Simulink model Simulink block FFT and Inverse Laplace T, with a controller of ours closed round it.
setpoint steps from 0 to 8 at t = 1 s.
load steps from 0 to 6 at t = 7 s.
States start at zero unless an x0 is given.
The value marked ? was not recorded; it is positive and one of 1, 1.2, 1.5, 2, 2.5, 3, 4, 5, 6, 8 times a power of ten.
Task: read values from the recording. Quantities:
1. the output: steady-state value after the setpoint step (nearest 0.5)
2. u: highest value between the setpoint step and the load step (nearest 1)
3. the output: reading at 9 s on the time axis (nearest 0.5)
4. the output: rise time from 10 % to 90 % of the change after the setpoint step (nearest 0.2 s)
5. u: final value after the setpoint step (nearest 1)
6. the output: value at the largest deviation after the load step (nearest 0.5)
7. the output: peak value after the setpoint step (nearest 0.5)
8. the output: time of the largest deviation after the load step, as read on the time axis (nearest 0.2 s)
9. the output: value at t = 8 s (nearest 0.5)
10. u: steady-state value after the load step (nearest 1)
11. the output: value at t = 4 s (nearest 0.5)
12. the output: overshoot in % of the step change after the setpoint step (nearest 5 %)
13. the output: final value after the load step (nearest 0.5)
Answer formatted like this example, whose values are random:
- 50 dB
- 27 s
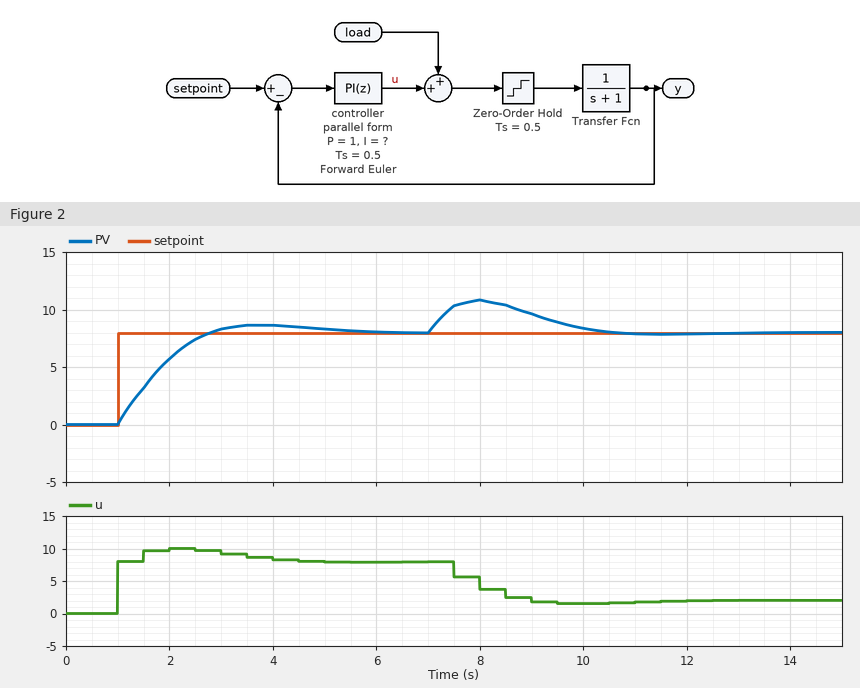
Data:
- 8.0
- 10
- 9.5
- 1.4 s
- 8
- 11.0
- 8.5
- 8.0 s
- 11.0
- 2
- 8.5
- 10 %
- 8.0
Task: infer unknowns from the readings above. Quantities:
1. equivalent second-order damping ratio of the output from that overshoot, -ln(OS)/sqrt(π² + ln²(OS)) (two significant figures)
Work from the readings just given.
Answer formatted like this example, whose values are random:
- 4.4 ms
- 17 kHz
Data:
- 0.59
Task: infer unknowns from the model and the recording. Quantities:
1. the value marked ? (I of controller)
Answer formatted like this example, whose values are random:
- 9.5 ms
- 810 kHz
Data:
- 1.2
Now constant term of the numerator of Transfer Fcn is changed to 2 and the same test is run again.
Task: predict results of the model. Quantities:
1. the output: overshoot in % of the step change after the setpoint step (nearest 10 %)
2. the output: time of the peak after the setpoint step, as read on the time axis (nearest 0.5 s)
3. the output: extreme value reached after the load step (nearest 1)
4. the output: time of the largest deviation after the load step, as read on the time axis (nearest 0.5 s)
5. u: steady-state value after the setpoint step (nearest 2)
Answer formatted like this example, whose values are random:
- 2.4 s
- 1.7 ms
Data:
- 20 %
- 2.5 s
- 13
- 7.5 s
- 4
